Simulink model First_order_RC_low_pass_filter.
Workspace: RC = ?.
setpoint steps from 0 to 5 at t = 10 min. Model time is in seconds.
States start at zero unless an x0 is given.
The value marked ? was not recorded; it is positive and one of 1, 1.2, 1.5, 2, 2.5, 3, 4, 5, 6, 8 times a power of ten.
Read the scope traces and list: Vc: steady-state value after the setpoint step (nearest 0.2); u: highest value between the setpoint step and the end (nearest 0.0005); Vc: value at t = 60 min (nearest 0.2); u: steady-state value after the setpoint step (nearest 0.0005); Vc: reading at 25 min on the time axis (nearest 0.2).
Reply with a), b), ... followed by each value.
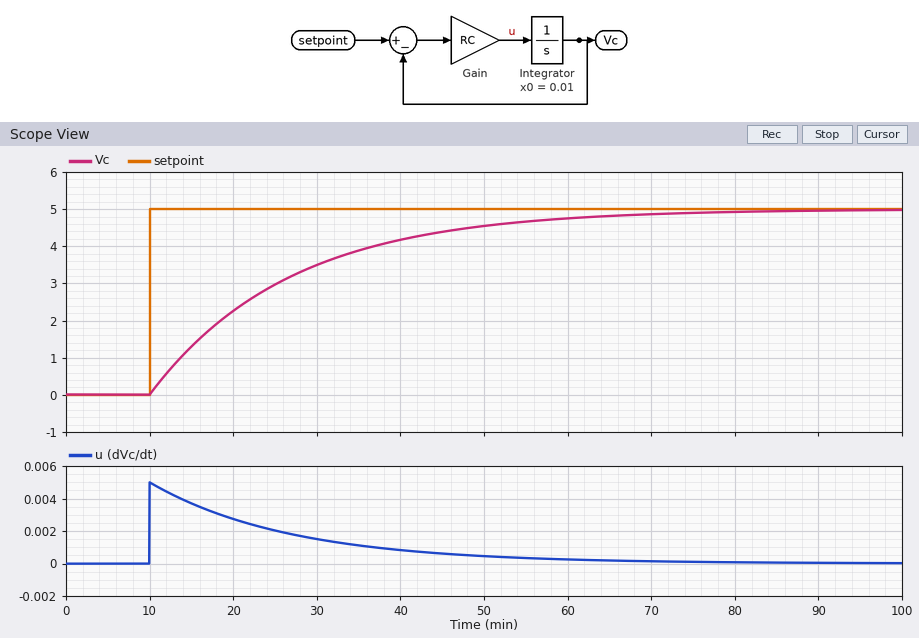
a) 5.0
b) 0.0050
c) 4.8
d) 0.0000
e) 3.0
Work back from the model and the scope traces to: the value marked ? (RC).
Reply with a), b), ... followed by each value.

a) 0.001
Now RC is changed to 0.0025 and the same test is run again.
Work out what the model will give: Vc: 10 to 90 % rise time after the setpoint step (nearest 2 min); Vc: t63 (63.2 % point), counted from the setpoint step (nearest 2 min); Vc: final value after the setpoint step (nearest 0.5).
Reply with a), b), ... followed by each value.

a) 14 min
b) 6 min
c) 5.0
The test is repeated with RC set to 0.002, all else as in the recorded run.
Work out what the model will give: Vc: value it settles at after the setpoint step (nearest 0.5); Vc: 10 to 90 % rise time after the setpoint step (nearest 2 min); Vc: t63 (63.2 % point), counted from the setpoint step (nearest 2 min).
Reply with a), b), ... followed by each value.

a) 5.0
b) 18 min
c) 8 min
